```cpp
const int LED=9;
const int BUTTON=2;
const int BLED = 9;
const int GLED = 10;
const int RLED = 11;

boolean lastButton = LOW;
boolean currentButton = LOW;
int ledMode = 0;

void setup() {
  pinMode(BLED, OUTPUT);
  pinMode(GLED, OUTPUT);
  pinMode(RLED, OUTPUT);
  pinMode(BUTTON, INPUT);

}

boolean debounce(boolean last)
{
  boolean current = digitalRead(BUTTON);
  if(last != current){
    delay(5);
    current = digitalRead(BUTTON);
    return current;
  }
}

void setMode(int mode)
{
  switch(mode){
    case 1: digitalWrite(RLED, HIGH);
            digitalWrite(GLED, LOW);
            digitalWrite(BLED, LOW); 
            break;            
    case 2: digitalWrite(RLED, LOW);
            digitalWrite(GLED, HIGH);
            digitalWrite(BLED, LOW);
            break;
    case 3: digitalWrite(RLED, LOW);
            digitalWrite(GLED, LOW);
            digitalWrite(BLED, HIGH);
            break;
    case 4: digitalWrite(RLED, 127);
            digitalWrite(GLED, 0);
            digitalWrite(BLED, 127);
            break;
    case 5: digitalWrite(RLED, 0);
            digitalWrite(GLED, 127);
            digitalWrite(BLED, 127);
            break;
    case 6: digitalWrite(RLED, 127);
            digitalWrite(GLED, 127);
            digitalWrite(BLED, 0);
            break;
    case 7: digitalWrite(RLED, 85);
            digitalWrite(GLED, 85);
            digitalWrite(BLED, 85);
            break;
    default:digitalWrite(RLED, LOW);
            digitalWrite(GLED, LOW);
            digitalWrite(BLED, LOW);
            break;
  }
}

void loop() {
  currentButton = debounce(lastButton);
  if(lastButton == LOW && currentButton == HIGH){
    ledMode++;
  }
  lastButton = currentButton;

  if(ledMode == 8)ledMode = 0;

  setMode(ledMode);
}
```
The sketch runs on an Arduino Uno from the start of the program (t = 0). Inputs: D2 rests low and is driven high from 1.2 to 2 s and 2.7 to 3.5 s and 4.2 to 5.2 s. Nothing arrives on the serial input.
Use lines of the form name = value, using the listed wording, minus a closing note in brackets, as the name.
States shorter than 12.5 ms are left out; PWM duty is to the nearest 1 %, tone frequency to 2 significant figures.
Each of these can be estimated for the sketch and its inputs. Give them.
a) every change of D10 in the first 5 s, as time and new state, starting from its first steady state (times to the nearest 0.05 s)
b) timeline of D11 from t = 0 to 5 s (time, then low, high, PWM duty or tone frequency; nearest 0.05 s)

every change of D10 in the first 5 s, as time and new state, starting from its first steady state = 0 s low; 2.7 s high; 4.2 s low
timeline of D11 from t = 0 to 5 s = 0 s low; 1.2 s high; 2.7 s low
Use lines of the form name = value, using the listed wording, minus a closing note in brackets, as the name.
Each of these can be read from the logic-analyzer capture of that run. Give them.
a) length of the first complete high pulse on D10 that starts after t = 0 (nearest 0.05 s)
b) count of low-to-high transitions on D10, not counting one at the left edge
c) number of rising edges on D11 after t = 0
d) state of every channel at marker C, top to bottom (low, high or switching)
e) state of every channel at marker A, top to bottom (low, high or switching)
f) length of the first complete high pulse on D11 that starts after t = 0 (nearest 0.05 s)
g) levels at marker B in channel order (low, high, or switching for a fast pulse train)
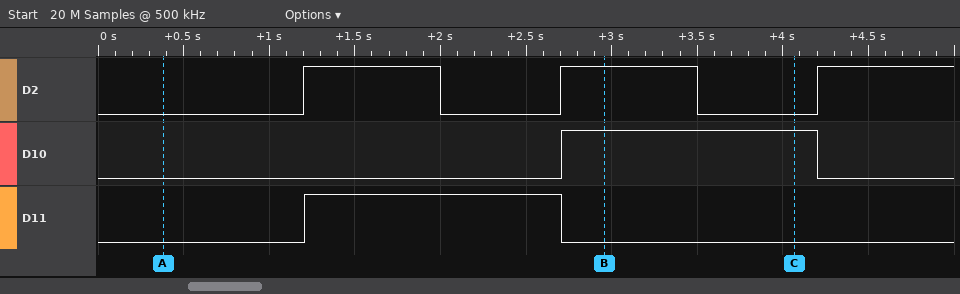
length of the first complete high pulse on D10 that starts after t = 0 = 1.50 s
count of low-to-high transitions on D10, not counting one at the left edge = 1
number of rising edges on D11 after t = 0 = 1
state of every channel at marker C, top to bottom = D2 low, D10 high, D11 low
state of every channel at marker A, top to bottom = D2 low, D10 low, D11 low
length of the first complete high pulse on D11 that starts after t = 0 = 1.50 s
levels at marker B in channel order = D2 high, D10 high, D11 low
